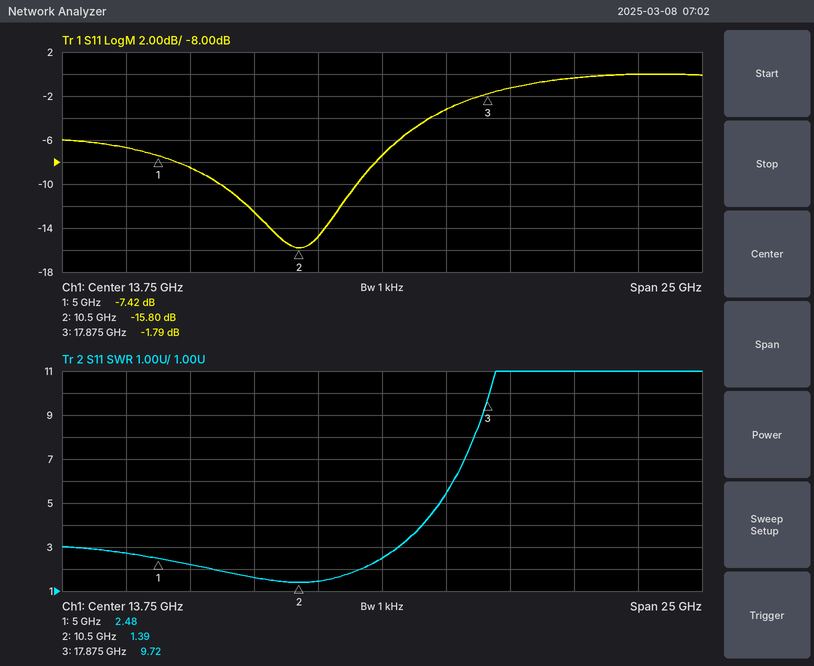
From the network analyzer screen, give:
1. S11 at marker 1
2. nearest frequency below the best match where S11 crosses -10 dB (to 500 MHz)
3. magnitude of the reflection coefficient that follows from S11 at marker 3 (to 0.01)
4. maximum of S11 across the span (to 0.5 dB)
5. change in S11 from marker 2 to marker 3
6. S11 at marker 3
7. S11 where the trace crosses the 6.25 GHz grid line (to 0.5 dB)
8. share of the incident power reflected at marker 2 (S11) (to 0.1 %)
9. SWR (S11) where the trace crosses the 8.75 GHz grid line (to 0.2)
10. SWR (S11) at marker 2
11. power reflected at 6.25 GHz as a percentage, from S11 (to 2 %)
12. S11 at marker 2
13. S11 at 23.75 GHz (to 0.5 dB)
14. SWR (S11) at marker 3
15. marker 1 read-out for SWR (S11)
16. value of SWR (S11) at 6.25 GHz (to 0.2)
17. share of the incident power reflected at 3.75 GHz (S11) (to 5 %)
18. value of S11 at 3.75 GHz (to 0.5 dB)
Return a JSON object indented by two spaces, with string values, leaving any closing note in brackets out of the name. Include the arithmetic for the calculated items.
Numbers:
{
  "S11 at marker 1": "-7.42 dB",
  "nearest frequency below the best match where S11 crosses -10 dB": "7.5 GHz",
  "magnitude of the reflection coefficient that follows from S11 at marker 3": "10^(-1.79/20) ≈ 0.81",
  "maximum of S11 across the span": "0.0 dB",
  "change in S11 from marker 2 to marker 3": "-1.79 − (-15.8) = 14.01 dB",
  "S11 at marker 3": "-1.79 dB",
  "S11 where the trace crosses the 6.25 GHz grid line": "-8.5 dB",
  "share of the incident power reflected at marker 2 (S11)": "10^(-15.8/10) ≈ 2.6 %",
  "SWR (S11) where the trace crosses the 8.75 GHz grid line": "1.6",
  "SWR (S11) at marker 2": "1.39",
  "power reflected at 6.25 GHz as a percentage, from S11": "10^(-8.5/10) ≈ 14 %",
  "S11 at marker 2": "-15.80 dB",
  "S11 at 23.75 GHz": "0.0 dB",
  "SWR (S11) at marker 3": "9.72",
  "marker 1 read-out for SWR": "2.48",
  "value of SWR (S11) at 6.25 GHz": "2.2",
  "share of the incident power reflected at 3.75 GHz (S11)": "10^(-6.5/10) ≈ 22.4 %, so 20 % to the nearest 5 %",
  "value of S11 at 3.75 GHz": "-6.5 dB"
}
